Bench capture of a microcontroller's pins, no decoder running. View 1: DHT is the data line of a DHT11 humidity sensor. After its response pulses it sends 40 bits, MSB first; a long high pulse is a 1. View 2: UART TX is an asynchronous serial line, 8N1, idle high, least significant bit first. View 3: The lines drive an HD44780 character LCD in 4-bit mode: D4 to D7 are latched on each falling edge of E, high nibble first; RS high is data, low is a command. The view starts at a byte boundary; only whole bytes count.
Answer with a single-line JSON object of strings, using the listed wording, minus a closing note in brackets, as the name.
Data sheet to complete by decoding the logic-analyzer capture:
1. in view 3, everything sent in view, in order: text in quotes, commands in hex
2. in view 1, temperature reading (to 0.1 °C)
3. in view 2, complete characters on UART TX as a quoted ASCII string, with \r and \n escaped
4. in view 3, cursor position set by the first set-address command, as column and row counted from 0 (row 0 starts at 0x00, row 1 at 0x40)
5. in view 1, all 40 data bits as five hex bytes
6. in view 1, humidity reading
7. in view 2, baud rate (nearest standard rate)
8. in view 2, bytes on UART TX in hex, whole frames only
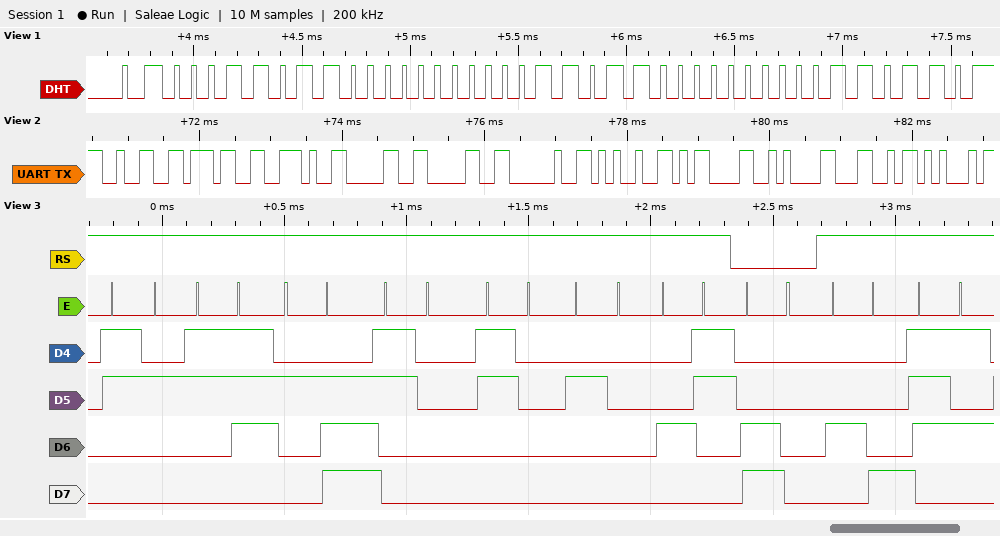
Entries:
{"in view 3, everything sent in view, in order: text in quotes, commands in hex": "\"27.00 C\" 0xC0 \"Hu\"", "in view 1, temperature reading": "27.0 °C", "in view 2, complete characters on UART TX as a quoted ASCII string, with \\r and \\n escaped": "\"27.00 %\\r\\nLE\"", "in view 3, cursor position set by the first set-address command, as column and row counted from 0": "column 0, row 1", "in view 1, all 40 data bits as five hex bytes": "1B 00 1B 00 36", "in view 1, humidity reading": "27 %", "in view 2, baud rate": "9600 baud", "in view 2, bytes on UART TX in hex, whole frames only": "32 37 2E 30 30 20 25 0D 0A 4C 45"}
